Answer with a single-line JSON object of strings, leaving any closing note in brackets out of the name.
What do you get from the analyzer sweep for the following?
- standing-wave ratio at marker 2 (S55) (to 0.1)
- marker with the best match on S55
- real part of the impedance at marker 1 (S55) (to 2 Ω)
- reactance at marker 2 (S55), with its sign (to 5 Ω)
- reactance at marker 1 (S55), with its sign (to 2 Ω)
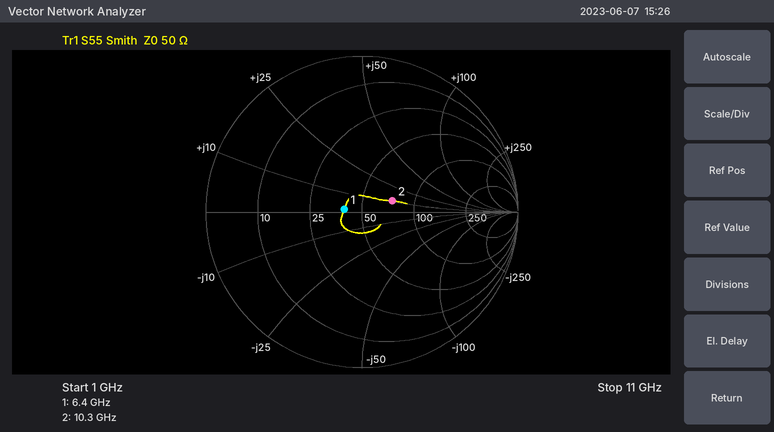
{"standing-wave ratio at marker 2 (S55)": "1.5", "marker with the best match on S55": "marker 1", "real part of the impedance at marker 1 (S55)": "40 Ω", "reactance at marker 2 (S55), with its sign": "+10 Ω", "reactance at marker 1 (S55), with its sign": "+2 Ω"}
